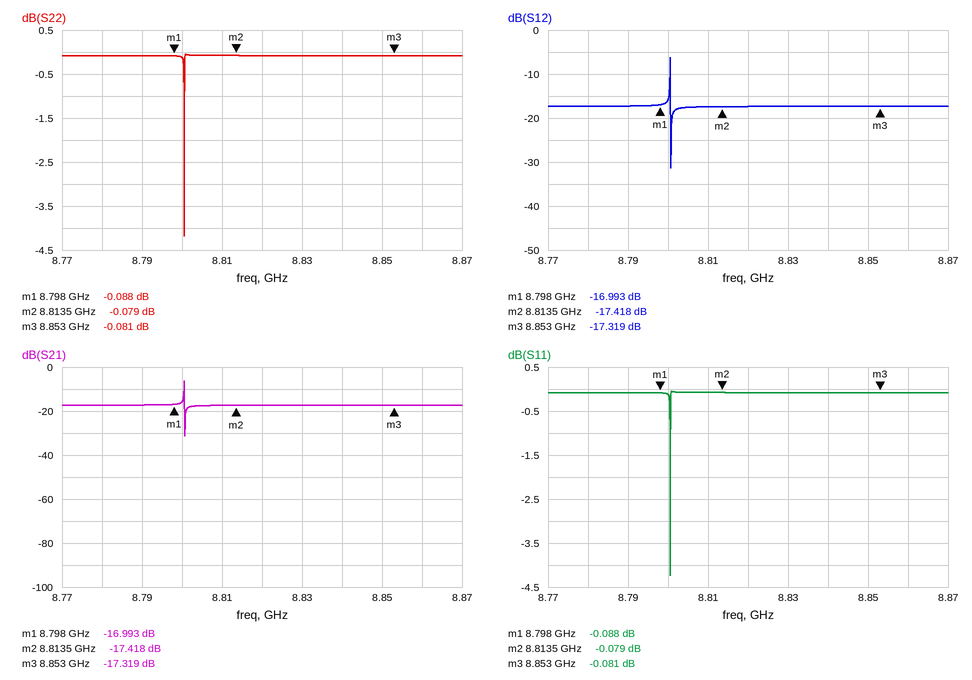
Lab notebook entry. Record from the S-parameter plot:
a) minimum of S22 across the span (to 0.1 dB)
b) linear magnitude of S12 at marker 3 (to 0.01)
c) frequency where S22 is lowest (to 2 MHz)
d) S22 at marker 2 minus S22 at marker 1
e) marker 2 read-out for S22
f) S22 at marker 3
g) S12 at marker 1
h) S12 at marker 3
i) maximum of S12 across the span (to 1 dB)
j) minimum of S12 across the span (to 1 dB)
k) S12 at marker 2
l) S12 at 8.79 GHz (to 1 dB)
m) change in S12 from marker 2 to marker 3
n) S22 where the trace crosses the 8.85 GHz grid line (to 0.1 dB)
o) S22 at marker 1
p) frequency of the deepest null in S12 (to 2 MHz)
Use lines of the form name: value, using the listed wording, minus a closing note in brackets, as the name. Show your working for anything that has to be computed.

minimum of S22 across the span: -4.2 dB
linear magnitude of S12 at marker 3: 10^(-17.319/20) ≈ 0.14
frequency where S22 is lowest: 8.800 GHz
S22 at marker 2 minus S22 at marker 1: -0.079 − (-0.088) = 0.009 dB
marker 2 read-out for S22: -0.079 dB
S22 at marker 3: -0.081 dB
S12 at marker 1: -16.993 dB
S12 at marker 3: -17.319 dB
maximum of S12 across the span: -6 dB
minimum of S12 across the span: -31 dB
S12 at marker 2: -17.418 dB
S12 at 8.79 GHz: -17 dB
change in S12 from marker 2 to marker 3: -17.319 − (-17.418) = 0.099 dB
S22 where the trace crosses the 8.85 GHz grid line: -0.1 dB
S22 at marker 1: -0.088 dB
frequency of the deepest null in S12: 8.800 GHz
